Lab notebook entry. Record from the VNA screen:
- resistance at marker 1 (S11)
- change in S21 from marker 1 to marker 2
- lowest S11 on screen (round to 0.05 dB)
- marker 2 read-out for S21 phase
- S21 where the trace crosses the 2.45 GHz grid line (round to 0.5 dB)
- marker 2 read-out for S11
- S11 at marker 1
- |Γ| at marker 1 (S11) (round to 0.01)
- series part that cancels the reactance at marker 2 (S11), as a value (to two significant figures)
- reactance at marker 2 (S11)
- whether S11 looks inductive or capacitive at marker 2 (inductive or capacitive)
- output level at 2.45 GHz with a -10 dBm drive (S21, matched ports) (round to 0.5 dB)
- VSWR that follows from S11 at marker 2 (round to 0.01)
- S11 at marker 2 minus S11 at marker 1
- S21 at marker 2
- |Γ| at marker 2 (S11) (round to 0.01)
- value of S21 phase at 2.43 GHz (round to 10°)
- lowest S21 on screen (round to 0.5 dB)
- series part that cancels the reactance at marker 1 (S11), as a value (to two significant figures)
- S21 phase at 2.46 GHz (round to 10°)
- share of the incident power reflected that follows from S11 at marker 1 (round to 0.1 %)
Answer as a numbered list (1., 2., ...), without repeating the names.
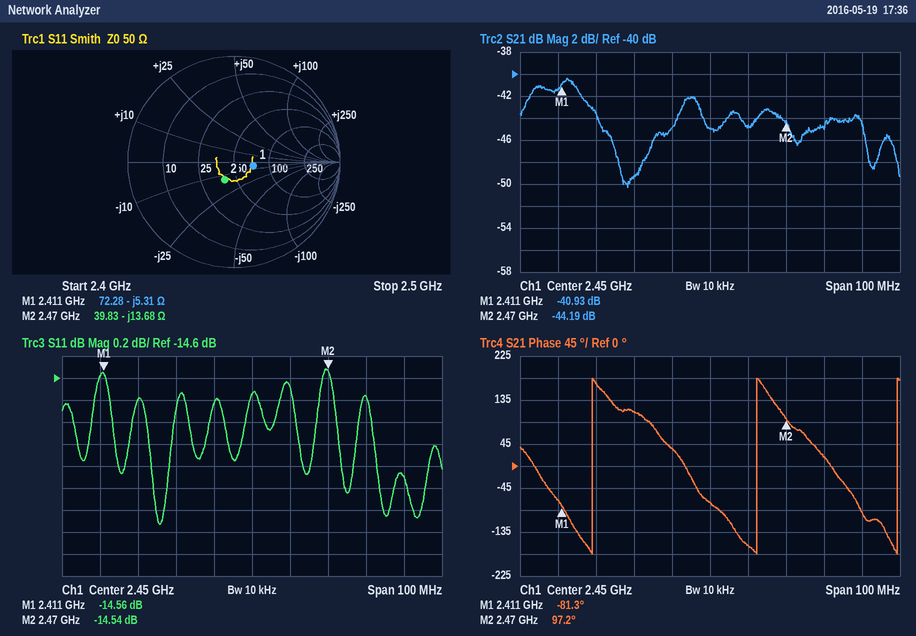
1. 72.28 Ω
2. -3.26 dB
3. -15.95 dB
4. 97.2°
5. -45.0 dB
6. -14.54 dB
7. -14.56 dB
8. 0.19
9. 880 pH
10. -13.68 Ω
11. capacitive
12. -55.0 dBm
13. 1.46
14. 0.02 dB
15. -44.19 dB
16. 0.19
17. 110°
18. -50.5 dB
19. 350 pH
20. -160°
21. 3.5 %
